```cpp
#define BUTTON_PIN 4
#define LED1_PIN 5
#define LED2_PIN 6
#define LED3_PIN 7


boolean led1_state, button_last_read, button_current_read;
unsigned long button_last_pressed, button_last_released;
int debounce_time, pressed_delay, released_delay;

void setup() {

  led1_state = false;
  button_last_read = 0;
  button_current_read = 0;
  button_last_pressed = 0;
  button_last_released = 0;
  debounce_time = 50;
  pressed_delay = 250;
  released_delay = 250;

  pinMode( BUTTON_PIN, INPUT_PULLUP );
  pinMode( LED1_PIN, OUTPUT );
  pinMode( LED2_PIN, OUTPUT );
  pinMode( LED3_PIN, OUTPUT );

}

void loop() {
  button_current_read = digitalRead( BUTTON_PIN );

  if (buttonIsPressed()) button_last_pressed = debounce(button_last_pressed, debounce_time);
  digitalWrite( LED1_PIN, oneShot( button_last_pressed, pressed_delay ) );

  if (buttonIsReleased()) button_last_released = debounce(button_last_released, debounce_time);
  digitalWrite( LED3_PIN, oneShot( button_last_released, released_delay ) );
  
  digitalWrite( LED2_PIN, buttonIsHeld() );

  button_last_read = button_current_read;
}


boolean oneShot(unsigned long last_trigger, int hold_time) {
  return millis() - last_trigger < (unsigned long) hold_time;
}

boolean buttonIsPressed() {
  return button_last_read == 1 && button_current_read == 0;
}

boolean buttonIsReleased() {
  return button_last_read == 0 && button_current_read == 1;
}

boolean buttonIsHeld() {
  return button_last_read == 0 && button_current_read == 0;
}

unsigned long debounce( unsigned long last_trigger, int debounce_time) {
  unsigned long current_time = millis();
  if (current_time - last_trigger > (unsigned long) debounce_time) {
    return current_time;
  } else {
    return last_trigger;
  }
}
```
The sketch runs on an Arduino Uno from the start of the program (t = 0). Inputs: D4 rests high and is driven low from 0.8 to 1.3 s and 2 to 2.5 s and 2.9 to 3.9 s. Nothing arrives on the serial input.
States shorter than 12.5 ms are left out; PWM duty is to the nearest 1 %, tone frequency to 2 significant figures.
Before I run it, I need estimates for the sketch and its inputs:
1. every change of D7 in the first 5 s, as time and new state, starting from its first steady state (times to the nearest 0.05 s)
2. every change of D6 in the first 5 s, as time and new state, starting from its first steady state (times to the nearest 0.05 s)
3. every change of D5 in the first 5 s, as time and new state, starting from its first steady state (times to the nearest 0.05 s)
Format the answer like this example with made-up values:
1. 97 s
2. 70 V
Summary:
1. 0 s high; 0.25 s low; 1.3 s high; 1.55 s low; 2.5 s high; 2.75 s low; 3.9 s high; 4.15 s low
2. 0 s low; 0.8 s high; 1.3 s low; 2 s high; 2.5 s low; 2.9 s high; 3.9 s low
3. 0 s high; 0.25 s low; 0.8 s high; 1.05 s low; 2 s high; 2.25 s low; 2.9 s high; 3.15 s low
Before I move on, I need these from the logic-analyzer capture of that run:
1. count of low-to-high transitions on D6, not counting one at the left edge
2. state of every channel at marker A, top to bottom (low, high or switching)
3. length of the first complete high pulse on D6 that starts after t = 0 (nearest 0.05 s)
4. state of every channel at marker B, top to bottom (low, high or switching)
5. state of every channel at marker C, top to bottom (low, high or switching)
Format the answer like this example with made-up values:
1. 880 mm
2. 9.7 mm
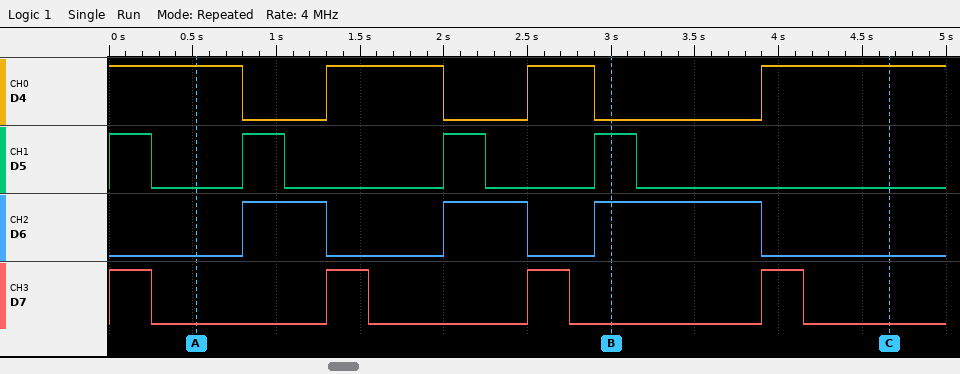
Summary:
1. 3
2. D4 high, D5 low, D6 low, D7 low
3. 0.50 s
4. D4 low, D5 high, D6 high, D7 low
5. D4 high, D5 low, D6 low, D7 low
